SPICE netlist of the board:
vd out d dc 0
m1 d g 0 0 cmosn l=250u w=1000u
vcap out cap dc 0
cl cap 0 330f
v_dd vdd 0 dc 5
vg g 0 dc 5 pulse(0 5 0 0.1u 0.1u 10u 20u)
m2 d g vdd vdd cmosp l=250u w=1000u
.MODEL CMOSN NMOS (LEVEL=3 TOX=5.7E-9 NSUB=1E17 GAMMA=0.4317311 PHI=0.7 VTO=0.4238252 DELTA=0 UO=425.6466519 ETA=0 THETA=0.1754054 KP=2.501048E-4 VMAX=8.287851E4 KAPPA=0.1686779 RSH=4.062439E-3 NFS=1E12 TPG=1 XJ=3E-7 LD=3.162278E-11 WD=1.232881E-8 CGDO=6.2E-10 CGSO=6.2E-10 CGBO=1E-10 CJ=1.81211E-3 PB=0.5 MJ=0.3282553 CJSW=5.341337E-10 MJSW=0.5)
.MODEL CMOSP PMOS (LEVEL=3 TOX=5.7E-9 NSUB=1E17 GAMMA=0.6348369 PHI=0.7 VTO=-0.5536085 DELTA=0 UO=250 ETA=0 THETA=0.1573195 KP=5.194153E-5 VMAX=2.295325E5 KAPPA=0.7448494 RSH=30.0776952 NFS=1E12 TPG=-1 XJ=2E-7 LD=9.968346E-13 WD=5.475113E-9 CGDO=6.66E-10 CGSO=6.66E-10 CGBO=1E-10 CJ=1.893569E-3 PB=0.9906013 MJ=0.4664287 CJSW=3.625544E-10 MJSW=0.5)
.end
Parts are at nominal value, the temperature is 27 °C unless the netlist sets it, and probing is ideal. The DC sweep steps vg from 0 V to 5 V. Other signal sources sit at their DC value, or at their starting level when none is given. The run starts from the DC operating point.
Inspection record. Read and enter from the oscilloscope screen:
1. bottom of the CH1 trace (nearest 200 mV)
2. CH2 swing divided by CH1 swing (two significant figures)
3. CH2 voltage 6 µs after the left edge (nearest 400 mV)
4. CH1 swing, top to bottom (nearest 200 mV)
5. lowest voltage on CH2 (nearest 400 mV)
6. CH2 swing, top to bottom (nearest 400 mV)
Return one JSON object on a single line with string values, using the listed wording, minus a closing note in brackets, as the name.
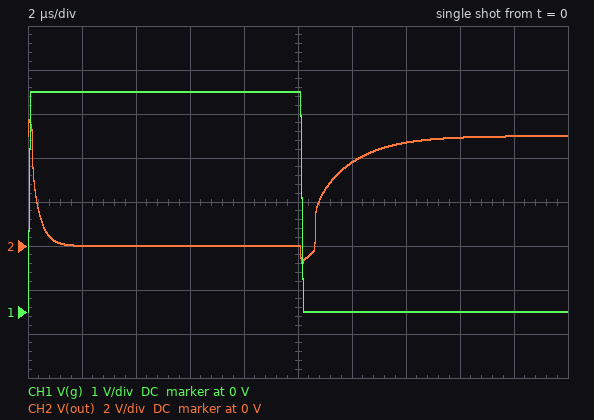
{"bottom of the CH1 trace": "0 V", "CH2 swing divided by CH1 swing": "1.3", "CH2 voltage 6 µs after the left edge": "0 V", "CH1 swing, top to bottom": "5.0 V", "lowest voltage on CH2": "-800 mV", "CH2 swing, top to bottom": "6.4 V"}
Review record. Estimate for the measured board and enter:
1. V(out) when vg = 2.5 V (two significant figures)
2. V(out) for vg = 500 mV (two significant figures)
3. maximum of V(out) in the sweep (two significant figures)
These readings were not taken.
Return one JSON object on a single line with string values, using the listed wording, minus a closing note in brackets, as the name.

{"V(out) when vg = 2.5 V": "170 mV", "V(out) for vg = 500 mV": "5.0 V", "maximum of V(out) in the sweep": "5.0 V"}
